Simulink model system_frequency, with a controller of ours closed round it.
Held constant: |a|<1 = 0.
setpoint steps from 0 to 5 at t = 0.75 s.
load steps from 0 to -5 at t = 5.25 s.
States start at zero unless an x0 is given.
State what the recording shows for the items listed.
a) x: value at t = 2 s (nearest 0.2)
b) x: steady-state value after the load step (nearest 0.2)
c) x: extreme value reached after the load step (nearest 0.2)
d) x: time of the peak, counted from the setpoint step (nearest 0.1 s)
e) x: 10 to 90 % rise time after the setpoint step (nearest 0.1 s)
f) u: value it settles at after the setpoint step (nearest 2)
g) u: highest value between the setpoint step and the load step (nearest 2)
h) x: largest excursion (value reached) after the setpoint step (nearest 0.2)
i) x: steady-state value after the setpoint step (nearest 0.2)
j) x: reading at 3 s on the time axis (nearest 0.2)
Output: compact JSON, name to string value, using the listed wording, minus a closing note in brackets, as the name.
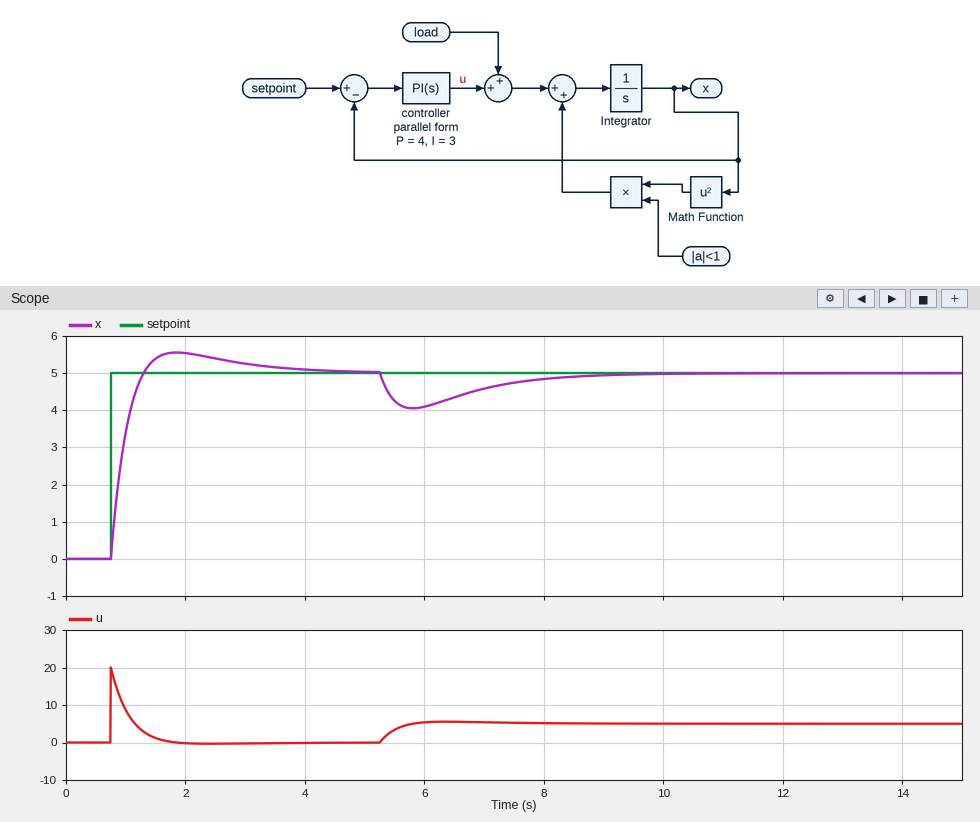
{"x: value at t = 2 s": "5.6", "x: steady-state value after the load step": "5.0", "x: extreme value reached after the load step": "4.0", "x: time of the peak, counted from the setpoint step": "1.1 s", "x: 10 to 90 % rise time after the setpoint step": "0.4 s", "u: value it settles at after the setpoint step": "0", "u: highest value between the setpoint step and the load step": "20", "x: largest excursion (value reached) after the setpoint step": "5.6", "x: steady-state value after the setpoint step": "5.0", "x: reading at 3 s on the time axis": "5.2"}
